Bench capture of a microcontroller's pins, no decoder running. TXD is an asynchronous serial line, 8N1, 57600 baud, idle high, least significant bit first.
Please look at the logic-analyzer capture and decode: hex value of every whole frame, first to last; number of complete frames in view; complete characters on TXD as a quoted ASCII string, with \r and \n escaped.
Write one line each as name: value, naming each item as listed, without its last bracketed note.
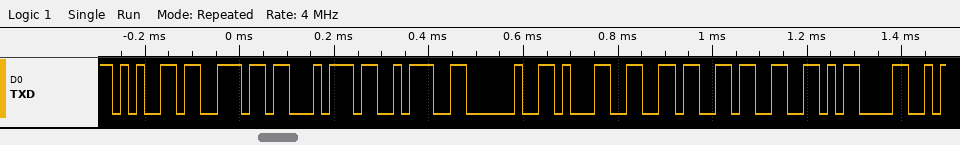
hex value of every whole frame, first to last: 0x65 0x6E 0x74 0x3A 0x20 0x31 0x36 0x33 0x0D
number of complete frames in view: 9
complete characters on TXD as a quoted ASCII string, with \r and \n escaped: "ent: 163\r"
